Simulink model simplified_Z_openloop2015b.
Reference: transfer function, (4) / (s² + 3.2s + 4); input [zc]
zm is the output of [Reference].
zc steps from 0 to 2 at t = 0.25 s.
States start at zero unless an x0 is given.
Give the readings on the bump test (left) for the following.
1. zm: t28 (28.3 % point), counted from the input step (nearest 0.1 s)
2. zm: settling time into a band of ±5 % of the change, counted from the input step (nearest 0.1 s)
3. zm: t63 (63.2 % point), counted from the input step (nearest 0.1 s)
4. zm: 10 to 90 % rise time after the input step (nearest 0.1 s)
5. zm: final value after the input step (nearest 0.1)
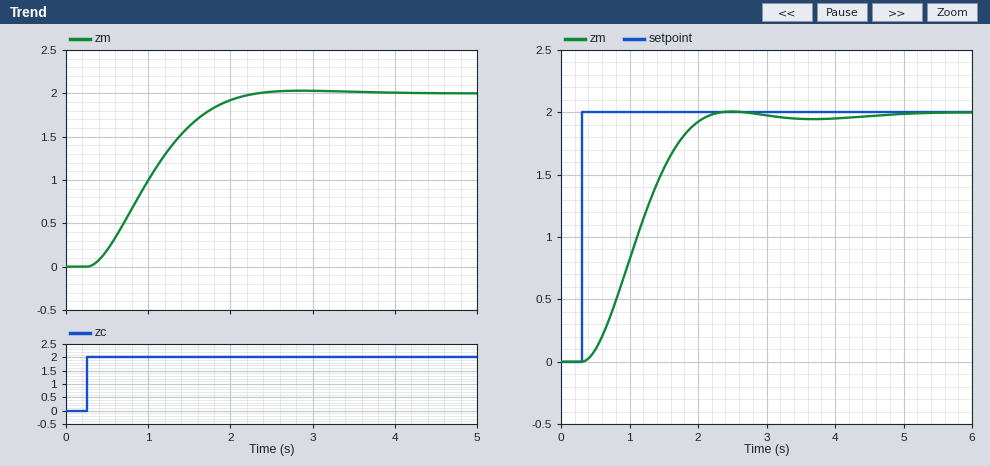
0.5 s
1.7 s
0.9 s
1.2 s
2.0
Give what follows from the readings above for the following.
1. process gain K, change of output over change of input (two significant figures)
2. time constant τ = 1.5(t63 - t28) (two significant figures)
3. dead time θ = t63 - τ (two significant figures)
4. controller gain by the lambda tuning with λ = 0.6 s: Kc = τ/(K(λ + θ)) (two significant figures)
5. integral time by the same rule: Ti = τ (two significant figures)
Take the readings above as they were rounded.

1.0
0.60 s
0.30 s
0.67
0.60 s
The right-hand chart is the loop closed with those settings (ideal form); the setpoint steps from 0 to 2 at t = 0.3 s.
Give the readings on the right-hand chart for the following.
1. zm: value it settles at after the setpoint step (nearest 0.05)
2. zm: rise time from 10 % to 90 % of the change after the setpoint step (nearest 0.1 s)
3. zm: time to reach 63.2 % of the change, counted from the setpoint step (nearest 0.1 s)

2.00
1.2 s
1.0 s
